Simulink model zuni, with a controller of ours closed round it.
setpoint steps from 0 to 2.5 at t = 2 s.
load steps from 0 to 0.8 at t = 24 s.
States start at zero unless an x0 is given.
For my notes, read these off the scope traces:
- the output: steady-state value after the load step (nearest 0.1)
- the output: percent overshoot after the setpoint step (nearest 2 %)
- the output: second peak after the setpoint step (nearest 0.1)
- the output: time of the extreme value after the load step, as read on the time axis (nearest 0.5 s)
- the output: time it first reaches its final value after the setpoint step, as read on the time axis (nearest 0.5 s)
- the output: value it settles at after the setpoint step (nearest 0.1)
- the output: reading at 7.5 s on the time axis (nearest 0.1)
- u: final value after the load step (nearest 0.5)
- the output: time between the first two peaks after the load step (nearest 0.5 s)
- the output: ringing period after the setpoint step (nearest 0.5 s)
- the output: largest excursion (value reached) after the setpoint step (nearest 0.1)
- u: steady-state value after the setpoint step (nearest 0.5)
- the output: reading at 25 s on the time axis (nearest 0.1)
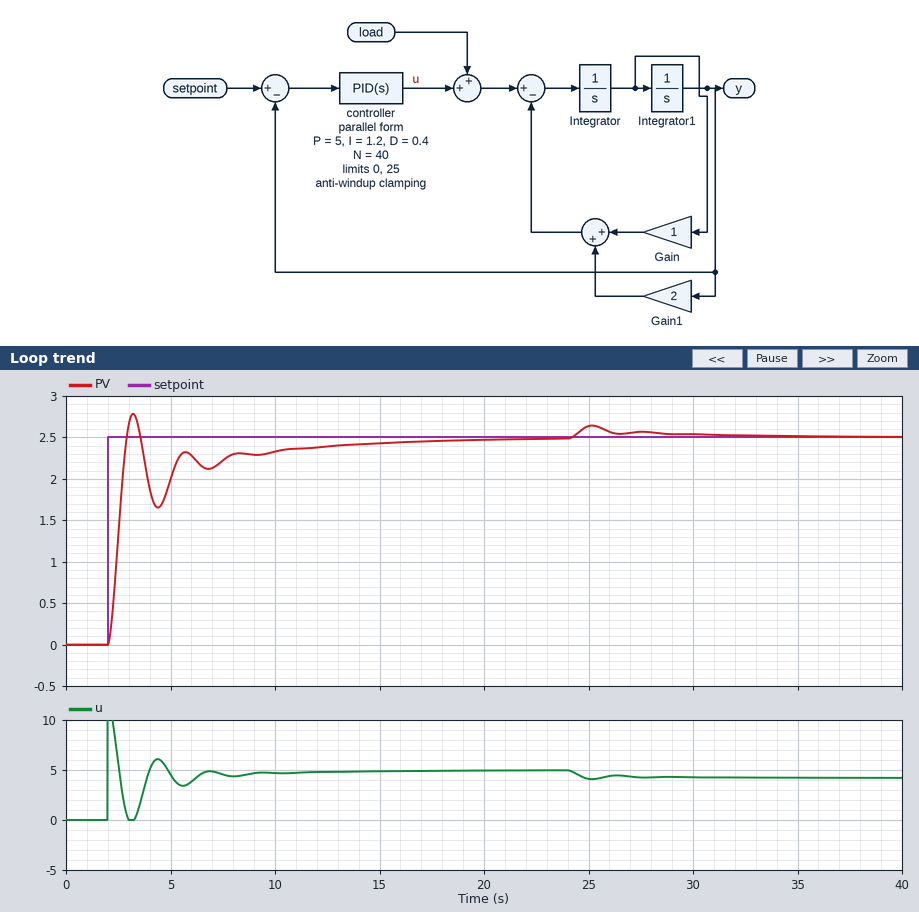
2.5
12 %
2.3
25.0 s
3.0 s
2.5
2.2
4.0
2.5 s
2.5 s
2.8
5.0
2.6
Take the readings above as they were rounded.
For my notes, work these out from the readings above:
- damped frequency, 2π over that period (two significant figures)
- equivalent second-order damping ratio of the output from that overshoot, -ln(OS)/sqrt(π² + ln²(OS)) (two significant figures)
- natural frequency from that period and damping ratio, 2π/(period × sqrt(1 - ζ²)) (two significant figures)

2.5 rad/s
0.56
3.0 rad/s
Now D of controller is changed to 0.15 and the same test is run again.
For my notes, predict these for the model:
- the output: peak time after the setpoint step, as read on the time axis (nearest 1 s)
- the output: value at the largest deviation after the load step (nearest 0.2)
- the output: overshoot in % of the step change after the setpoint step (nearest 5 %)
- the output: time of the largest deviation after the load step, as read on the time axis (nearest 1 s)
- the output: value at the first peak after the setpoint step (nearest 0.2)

3 s
2.6
20 %
25 s
3.0
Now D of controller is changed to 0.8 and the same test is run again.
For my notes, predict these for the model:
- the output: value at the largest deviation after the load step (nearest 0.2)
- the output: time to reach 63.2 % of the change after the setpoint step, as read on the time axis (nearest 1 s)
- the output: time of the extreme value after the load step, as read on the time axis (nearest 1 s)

2.6
3 s
25 s
